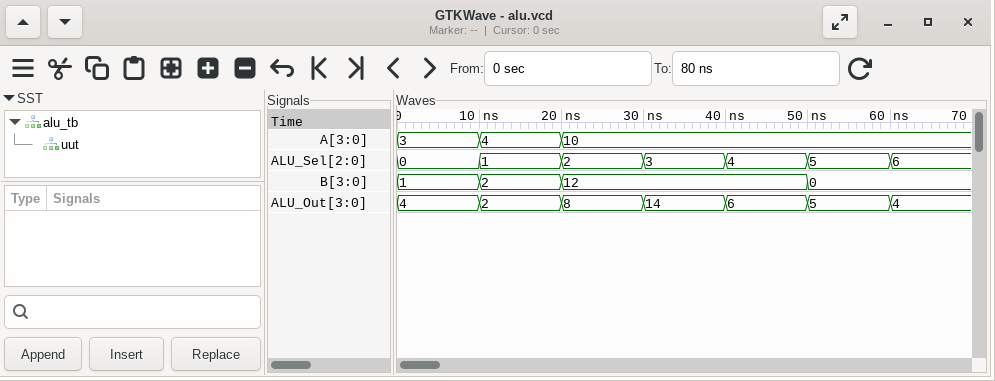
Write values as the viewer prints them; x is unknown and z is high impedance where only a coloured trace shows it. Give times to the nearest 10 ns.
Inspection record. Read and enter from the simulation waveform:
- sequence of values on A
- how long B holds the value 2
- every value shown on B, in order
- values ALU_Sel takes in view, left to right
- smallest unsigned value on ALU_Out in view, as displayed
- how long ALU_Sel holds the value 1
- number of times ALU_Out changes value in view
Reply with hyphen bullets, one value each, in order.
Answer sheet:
- 3, 4, 10
- 10 ns
- 1, 2, 12, 0
- 0, 1, 2, 3, 4, 5, 6
- 2
- 10 ns
- 6
